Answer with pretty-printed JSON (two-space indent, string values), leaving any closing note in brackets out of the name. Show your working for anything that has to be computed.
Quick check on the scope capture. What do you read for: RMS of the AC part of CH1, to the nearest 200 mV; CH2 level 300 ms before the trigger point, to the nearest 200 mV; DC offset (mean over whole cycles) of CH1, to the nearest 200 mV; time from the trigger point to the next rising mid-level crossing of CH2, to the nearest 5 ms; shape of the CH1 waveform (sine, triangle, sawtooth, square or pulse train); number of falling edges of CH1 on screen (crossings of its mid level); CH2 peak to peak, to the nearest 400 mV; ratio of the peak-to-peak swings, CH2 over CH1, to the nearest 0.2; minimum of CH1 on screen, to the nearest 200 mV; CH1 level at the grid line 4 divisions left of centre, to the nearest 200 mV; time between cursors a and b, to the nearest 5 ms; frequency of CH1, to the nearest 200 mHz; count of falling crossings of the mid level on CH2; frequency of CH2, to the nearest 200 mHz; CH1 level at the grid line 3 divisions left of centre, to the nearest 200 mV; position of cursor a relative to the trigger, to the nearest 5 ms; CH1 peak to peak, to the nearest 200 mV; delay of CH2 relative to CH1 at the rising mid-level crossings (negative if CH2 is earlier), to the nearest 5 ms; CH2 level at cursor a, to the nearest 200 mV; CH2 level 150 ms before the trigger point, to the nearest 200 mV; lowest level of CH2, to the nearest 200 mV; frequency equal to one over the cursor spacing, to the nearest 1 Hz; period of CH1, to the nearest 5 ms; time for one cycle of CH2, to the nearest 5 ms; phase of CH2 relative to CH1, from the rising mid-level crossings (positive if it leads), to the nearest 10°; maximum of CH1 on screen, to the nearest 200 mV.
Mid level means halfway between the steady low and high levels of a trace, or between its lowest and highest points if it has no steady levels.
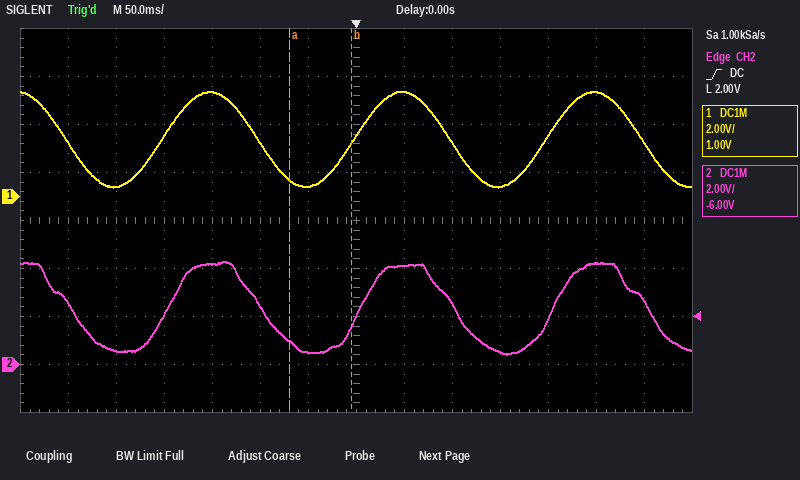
{
  "RMS of the AC part of CH1, to the nearest 200 mV": "4.0 V / (2√2) ≈ 1.4 V",
  "CH2 level 300 ms before the trigger point, to the nearest 200 mV": "2.6 V",
  "DC offset (mean over whole cycles) of CH1, to the nearest 200 mV": "(4.4 V + (400 mV)) / 2 ≈ 2.4 V",
  "time from the trigger point to the next rising mid-level crossing of CH2, to the nearest 5 ms": "5 ms",
  "shape of the CH1 waveform": "sine",
  "number of falling edges of CH1 on screen": "4",
  "CH2 peak to peak, to the nearest 400 mV": "4.0 V",
  "ratio of the peak-to-peak swings, CH2 over CH1, to the nearest 0.2": "4.0 V / 4.0 V ≈ 1.0",
  "minimum of CH1 on screen, to the nearest 200 mV": "400 mV",
  "CH1 level at the grid line 4 divisions left of centre, to the nearest 200 mV": "2.6 V",
  "time between cursors a and b, to the nearest 5 ms": "65 ms",
  "frequency of CH1, to the nearest 200 mHz": "1 / 200 ms ≈ 5.0 Hz",
  "count of falling crossings of the mid level on CH2": "4",
  "frequency of CH2, to the nearest 200 mHz": "1 / 200 ms ≈ 5.0 Hz",
  "CH1 level at the grid line 3 divisions left of centre, to the nearest 200 mV": "4.4 V",
  "position of cursor a relative to the trigger, to the nearest 5 ms": "-70 ms",
  "CH1 peak to peak, to the nearest 200 mV": "4.4 V − (400 mV) = 4.0 V",
  "delay of CH2 relative to CH1 at the rising mid-level crossings (negative if CH2 is earlier), to the nearest 5 ms": "+5 ms",
  "CH2 level at cursor a, to the nearest 200 mV": "1.0 V",
  "CH2 level 150 ms before the trigger point, to the nearest 200 mV": "4.2 V",
  "lowest level of CH2, to the nearest 200 mV": "400 mV",
  "frequency equal to one over the cursor spacing, to the nearest 1 Hz": "1 / 65 ms ≈ 15 Hz",
  "period of CH1, to the nearest 5 ms": "200 ms",
  "time for one cycle of CH2, to the nearest 5 ms": "200 ms",
  "phase of CH2 relative to CH1, from the rising mid-level crossings (positive if it leads), to the nearest 10°": "−360° × (+5 ms) / 200 ms ≈ -9.00°, so -10° to the nearest 10°",
  "maximum of CH1 on screen, to the nearest 200 mV": "4.4 V"
}
